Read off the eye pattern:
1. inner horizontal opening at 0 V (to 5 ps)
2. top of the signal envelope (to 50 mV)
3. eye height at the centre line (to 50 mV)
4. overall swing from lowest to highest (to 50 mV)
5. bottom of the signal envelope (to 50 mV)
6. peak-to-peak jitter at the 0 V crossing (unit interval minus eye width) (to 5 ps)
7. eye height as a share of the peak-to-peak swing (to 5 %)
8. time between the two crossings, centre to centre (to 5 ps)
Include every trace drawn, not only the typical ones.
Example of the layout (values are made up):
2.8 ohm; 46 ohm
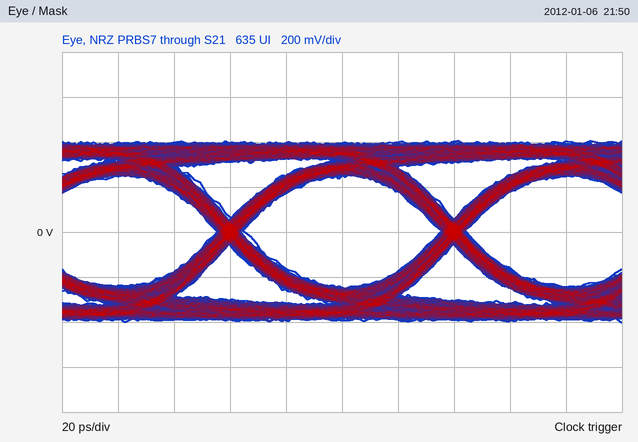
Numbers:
70 ps; 400 mV; 500 mV; 800 mV; -400 mV; 10 ps; 60 %; 80 ps
